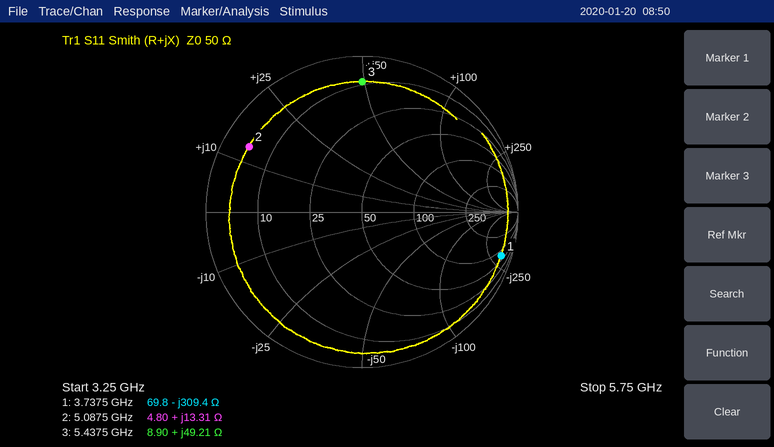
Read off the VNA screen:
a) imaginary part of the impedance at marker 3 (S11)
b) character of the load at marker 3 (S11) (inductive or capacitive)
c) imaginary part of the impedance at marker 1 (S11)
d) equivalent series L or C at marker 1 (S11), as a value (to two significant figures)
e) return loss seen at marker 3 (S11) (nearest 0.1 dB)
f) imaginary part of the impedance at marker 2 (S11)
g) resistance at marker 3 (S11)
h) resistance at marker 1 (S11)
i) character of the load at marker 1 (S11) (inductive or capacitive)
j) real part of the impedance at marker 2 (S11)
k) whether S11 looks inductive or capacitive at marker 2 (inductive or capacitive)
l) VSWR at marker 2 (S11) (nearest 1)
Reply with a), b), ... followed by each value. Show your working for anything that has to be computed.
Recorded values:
a) +49.21 Ω
b) inductive
c) -309.4 Ω
d) C = 1/(2π × 3.7375 GHz × 309.4 Ω) ≈ 138 fF, so 140 fF to two significant figures
e) 1.6 dB
f) +13.31 Ω
g) 8.90 Ω
h) 69.8 Ω
i) capacitive
j) 4.80 Ω
k) inductive
l) 11
